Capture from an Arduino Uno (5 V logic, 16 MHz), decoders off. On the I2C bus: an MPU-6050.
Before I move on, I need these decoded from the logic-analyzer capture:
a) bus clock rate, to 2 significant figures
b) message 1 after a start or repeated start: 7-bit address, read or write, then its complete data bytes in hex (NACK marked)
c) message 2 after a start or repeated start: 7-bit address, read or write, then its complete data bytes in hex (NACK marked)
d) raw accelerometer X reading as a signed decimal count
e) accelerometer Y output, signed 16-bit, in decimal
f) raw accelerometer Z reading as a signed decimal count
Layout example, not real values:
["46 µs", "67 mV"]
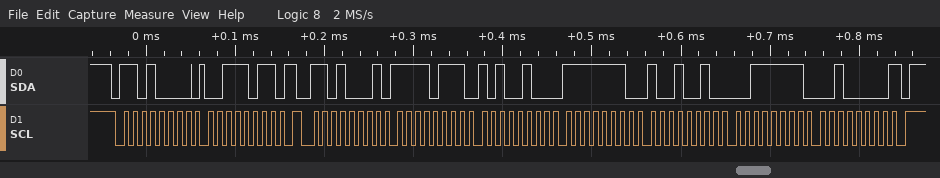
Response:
["100 kHz", "0x68 write: 3B", "0x68 read: F7 A4 FE 92 3F 20 NACK", "-2140", "-366", "16160"]
